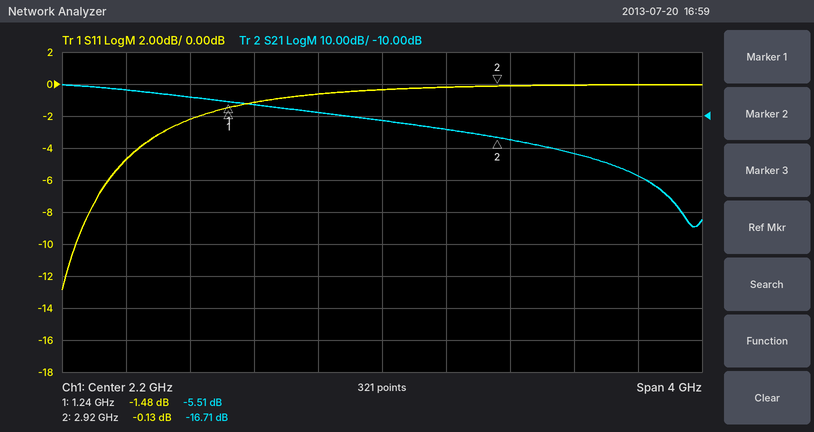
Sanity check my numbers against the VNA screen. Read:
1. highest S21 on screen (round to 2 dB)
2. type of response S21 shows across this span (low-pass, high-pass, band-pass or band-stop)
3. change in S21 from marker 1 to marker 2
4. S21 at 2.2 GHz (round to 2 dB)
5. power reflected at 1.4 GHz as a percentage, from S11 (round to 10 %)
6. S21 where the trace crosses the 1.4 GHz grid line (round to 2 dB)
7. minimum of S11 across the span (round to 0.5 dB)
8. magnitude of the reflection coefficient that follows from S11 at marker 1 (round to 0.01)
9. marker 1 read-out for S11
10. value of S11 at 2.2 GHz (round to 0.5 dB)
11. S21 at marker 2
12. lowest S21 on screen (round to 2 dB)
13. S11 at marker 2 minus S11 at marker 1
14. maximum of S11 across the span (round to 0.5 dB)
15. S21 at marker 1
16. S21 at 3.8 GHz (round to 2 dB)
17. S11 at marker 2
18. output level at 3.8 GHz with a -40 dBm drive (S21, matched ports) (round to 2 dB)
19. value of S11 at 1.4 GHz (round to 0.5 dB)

0 dB
low-pass
-11.20 dB
-12 dB
80 %
-6 dB
-13.0 dB
0.84
-1.48 dB
-0.5 dB
-16.71 dB
-44 dB
1.35 dB
0.0 dB
-5.51 dB
-28 dB
-0.13 dB
-68 dBm
-1.0 dB
